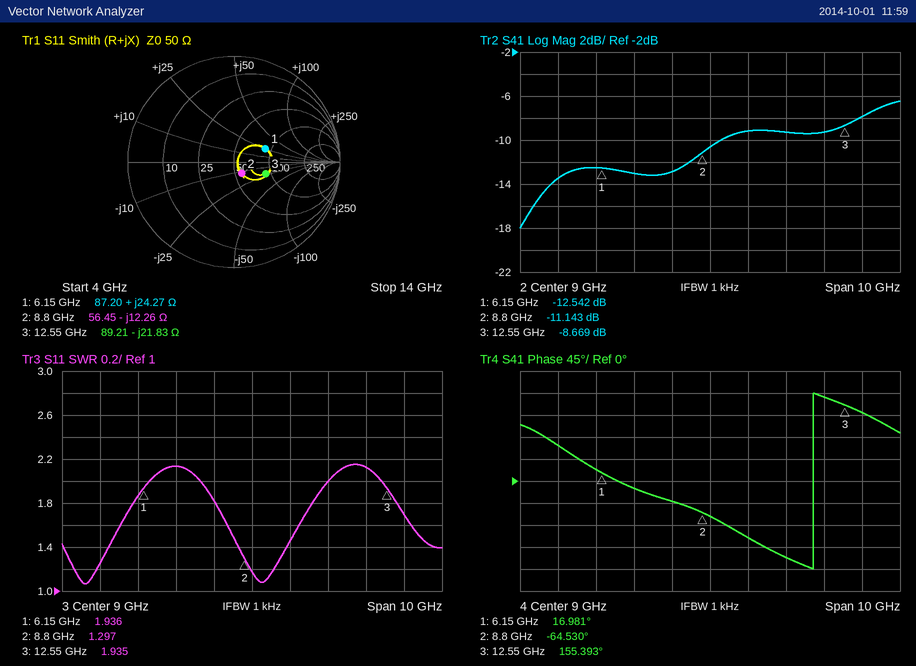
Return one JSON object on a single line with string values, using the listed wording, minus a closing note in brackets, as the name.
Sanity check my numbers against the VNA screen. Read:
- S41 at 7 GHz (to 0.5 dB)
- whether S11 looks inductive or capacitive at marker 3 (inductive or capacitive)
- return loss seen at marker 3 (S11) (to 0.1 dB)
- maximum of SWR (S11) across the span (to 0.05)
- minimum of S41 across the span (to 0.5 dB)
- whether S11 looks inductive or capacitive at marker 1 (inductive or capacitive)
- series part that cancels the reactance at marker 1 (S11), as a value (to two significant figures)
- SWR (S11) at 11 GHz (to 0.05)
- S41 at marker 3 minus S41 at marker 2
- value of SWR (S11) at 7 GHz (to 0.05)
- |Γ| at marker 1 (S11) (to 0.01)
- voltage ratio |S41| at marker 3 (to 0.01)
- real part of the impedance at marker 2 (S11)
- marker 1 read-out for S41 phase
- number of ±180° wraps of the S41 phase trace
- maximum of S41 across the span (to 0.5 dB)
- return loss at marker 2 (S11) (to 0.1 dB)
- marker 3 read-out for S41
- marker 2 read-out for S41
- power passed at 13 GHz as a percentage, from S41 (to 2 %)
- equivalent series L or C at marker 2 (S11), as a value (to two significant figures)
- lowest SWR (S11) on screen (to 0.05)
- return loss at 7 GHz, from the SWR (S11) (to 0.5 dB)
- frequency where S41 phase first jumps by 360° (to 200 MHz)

{"S41 at 7 GHz": "-13.0 dB", "whether S11 looks inductive or capacitive at marker 3": "capacitive", "return loss seen at marker 3 (S11)": "9.9 dB", "maximum of SWR (S11) across the span": "2.15", "minimum of S41 across the span": "-18.0 dB", "whether S11 looks inductive or capacitive at marker 1": "inductive", "series part that cancels the reactance at marker 1 (S11), as a value": "1.1 pF", "SWR (S11) at 11 GHz": "2.00", "S41 at marker 3 minus S41 at marker 2": "2.474 dB", "value of SWR (S11) at 7 GHz": "2.15", "|Γ| at marker 1 (S11)": "0.32", "voltage ratio |S41| at marker 3": "0.37", "real part of the impedance at marker 2": "56.45 Ω", "marker 1 read-out for S41 phase": "16.981°", "number of ±180° wraps of the S41 phase trace": "1", "maximum of S41 across the span": "-6.5 dB", "return loss at marker 2 (S11)": "17.8 dB", "marker 3 read-out for S41": "-8.669 dB", "marker 2 read-out for S41": "-11.143 dB", "power passed at 13 GHz as a percentage, from S41": "16 %", "equivalent series L or C at marker 2 (S11), as a value": "1.5 pF", "lowest SWR (S11) on screen": "1.05", "return loss at 7 GHz, from the SWR (S11)": "9.0 dB", "frequency where S41 phase first jumps by 360°": "11.8 GHz"}
